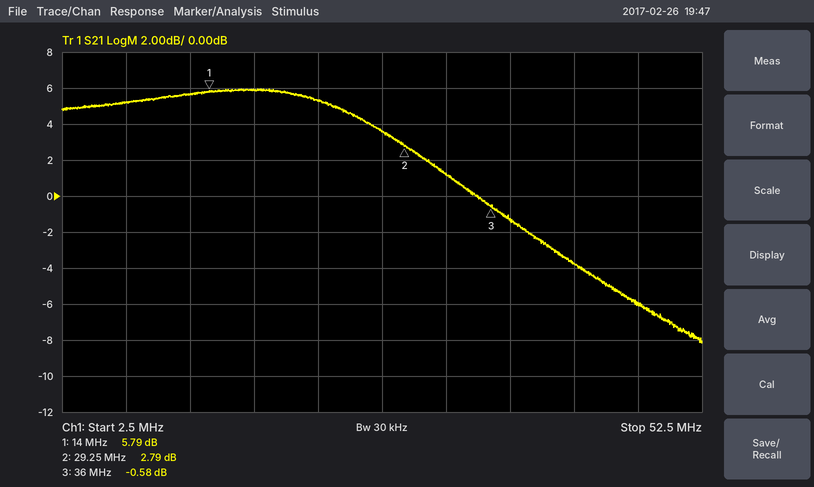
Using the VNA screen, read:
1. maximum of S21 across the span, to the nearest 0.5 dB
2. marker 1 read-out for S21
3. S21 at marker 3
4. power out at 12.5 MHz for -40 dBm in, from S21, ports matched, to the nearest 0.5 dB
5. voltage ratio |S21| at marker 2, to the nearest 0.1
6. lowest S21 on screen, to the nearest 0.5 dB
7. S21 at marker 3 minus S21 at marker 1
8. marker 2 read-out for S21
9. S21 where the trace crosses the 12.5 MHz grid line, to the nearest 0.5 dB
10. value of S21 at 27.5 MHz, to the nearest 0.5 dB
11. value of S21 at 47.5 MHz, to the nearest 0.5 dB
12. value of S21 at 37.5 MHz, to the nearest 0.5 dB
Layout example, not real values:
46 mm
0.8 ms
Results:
6.0 dB
5.79 dB
-0.58 dB
-34.5 dBm
1.4
-8.0 dB
-6.37 dB
2.79 dB
5.5 dB
3.5 dB
-6.0 dB
-1.5 dB
